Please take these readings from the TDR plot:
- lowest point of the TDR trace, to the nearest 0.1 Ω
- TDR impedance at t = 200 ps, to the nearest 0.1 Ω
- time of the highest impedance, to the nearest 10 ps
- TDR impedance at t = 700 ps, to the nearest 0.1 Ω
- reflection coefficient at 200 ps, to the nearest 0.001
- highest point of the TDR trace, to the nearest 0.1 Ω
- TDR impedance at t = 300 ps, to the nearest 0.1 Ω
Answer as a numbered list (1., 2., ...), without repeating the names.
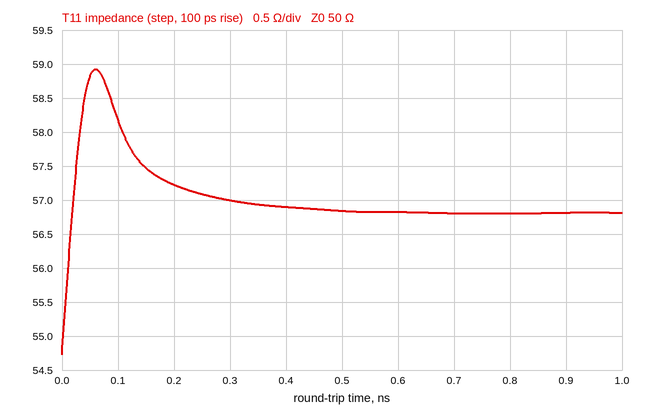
1. 54.7 Ω
2. 57.2 Ω
3. 60 ps
4. 56.8 Ω
5. +0.067
6. 58.9 Ω
7. 57.0 Ω
